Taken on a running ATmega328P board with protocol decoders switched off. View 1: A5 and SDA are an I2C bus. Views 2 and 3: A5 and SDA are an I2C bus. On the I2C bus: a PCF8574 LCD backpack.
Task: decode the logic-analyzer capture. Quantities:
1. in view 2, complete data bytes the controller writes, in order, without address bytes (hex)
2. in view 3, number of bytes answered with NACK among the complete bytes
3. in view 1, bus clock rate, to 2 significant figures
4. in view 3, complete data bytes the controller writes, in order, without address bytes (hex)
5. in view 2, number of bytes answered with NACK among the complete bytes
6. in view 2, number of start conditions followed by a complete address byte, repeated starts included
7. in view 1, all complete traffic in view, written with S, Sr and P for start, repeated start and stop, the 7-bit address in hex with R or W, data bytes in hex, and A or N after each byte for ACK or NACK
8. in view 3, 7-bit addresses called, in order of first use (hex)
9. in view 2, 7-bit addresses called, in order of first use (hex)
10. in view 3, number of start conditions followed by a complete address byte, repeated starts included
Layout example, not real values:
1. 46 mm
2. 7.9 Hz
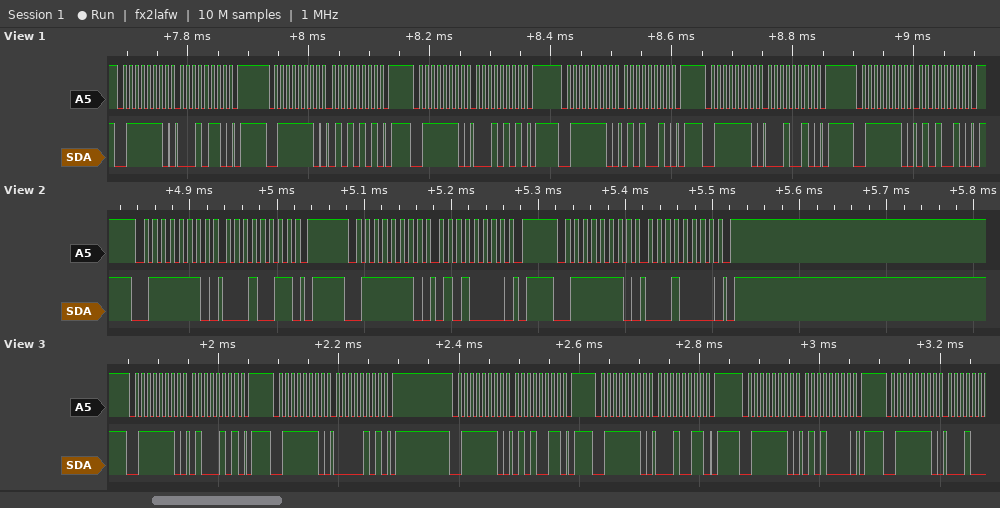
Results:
1. 13 50 10
2. 0
3. 100 kHz
4. 45 05 53 13 50
5. 0
6. 3
7. S 3FW A 16 A P S 3FW A 55 A P S 3FW A 15 A P S 3FW A 52 A P S 3FW A 12 A P S 3FW A 52 A P
8. 0x3F
9. 0x3F
10. 6
